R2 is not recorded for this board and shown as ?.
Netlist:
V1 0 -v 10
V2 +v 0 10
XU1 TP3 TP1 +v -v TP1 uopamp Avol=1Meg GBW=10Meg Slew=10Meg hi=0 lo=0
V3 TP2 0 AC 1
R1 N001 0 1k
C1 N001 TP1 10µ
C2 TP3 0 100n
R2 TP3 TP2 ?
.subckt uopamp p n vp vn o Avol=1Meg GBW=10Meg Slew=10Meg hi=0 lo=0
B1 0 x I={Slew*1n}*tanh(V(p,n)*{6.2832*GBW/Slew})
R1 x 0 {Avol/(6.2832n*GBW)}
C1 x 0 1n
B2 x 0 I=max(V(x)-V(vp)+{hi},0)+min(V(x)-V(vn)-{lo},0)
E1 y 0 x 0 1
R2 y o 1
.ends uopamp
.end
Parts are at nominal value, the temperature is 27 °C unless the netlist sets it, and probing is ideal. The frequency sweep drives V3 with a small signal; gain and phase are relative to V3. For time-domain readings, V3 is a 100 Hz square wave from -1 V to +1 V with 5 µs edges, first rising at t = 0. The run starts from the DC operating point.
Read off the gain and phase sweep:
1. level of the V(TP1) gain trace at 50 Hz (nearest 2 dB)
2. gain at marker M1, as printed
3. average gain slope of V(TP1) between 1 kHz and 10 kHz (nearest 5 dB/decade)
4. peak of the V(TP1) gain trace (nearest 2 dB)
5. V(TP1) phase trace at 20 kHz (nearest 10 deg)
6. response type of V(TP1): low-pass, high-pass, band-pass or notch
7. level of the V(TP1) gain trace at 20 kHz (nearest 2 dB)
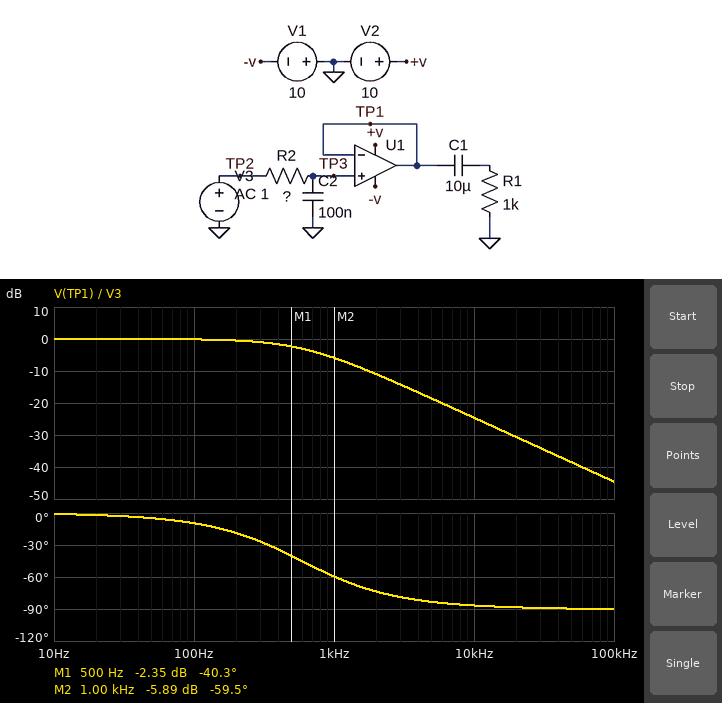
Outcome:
0 dB
-2.35 dB
-20 dB/decade
0 dB
-90 deg
low-pass
-30 dB
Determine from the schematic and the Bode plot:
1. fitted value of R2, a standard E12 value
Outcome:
2.7 kΩ
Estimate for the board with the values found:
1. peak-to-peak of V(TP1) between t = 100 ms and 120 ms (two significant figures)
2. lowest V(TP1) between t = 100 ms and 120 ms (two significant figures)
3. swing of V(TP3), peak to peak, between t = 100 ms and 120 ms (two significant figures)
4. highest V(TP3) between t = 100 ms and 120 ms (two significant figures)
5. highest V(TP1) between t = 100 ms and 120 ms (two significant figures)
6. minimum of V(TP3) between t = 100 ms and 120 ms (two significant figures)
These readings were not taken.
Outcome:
2.0 V
-1.0 V
2.0 V
1.0 V
1.0 V
-1.0 V
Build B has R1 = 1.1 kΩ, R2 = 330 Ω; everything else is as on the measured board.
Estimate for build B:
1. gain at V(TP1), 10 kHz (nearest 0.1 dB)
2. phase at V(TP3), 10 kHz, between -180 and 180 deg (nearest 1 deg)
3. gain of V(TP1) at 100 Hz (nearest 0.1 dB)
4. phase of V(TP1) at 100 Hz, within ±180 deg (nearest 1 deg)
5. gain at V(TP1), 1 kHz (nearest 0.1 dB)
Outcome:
-7.2 dB
-64 deg
0 dB
-1 deg
-0.2 dB
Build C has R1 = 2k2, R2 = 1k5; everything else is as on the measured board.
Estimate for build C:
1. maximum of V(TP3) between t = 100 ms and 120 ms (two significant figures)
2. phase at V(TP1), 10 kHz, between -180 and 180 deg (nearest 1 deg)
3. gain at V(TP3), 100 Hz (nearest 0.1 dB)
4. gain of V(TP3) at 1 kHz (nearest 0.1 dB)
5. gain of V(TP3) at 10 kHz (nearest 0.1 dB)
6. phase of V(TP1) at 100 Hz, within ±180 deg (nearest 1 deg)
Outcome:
1.0 V
-84 deg
0 dB
-2.8 dB
-19.5 dB
-5 deg
